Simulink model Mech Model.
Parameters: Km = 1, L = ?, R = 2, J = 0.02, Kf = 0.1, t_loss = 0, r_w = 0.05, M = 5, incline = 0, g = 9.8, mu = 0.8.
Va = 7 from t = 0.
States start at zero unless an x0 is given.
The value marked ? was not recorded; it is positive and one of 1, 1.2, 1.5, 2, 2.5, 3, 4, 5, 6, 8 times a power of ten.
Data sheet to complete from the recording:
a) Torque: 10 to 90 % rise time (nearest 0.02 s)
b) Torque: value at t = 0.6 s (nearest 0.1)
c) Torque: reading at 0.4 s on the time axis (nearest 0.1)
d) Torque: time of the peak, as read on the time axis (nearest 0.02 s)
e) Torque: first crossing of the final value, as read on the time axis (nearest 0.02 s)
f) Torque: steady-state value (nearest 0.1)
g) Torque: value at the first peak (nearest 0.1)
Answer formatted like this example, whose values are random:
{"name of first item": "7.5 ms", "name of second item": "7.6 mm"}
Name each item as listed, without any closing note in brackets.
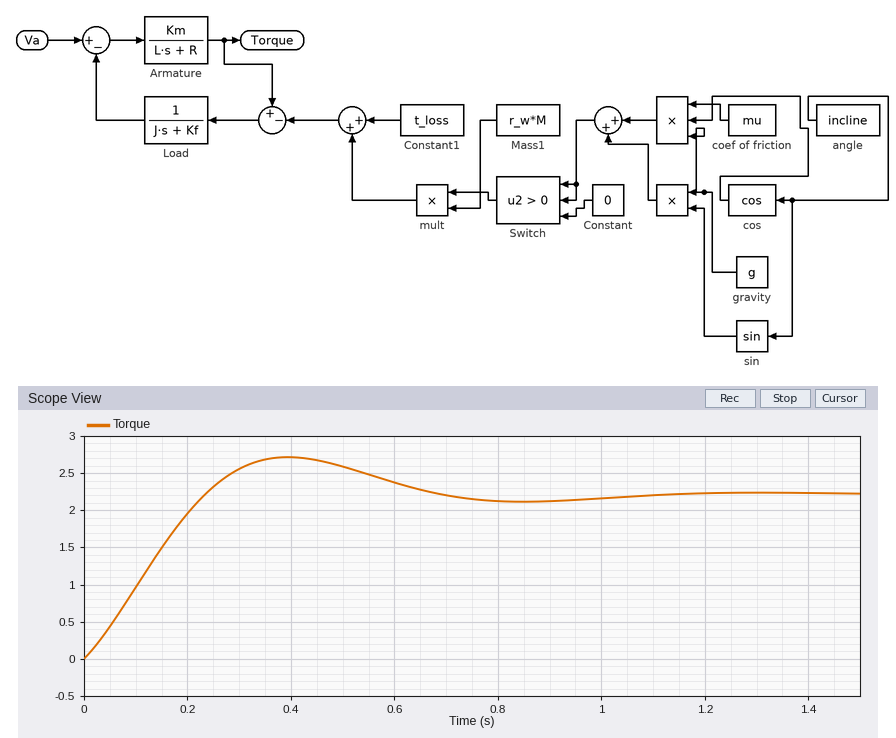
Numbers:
{"Torque: 10 to 90 % rise time": "0.18 s", "Torque: value at t = 0.6 s": "2.4", "Torque: reading at 0.4 s on the time axis": "2.7", "Torque: time of the peak, as read on the time axis": "0.40 s", "Torque: first crossing of the final value, as read on the time axis": "0.24 s", "Torque: steady-state value": "2.2", "Torque: value at the first peak": "2.7"}
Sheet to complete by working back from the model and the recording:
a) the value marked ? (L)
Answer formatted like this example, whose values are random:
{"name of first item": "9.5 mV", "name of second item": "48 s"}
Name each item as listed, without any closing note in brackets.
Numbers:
{"the value marked ?": "1"}
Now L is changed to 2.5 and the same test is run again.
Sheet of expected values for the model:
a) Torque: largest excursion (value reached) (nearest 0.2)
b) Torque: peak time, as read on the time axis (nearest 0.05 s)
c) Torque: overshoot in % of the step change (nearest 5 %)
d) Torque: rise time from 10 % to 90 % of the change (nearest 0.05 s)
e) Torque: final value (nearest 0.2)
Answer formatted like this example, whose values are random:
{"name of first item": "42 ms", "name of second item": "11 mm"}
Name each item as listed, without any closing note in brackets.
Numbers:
{"Torque: largest excursion (value reached)": "2.4", "Torque: peak time, as read on the time axis": "0.75 s", "Torque: overshoot in % of the step change": "10 %", "Torque: rise time from 10 % to 90 % of the change": "0.35 s", "Torque: final value": "2.2"}
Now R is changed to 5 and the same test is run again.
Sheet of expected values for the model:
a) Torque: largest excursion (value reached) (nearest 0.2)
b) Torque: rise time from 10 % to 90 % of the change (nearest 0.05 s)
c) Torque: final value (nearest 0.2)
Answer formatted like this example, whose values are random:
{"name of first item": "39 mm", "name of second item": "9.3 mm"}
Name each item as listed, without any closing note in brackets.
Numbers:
{"Torque: largest excursion (value reached)": "2.0", "Torque: rise time from 10 % to 90 % of the change": "0.20 s", "Torque: final value": "1.8"}
